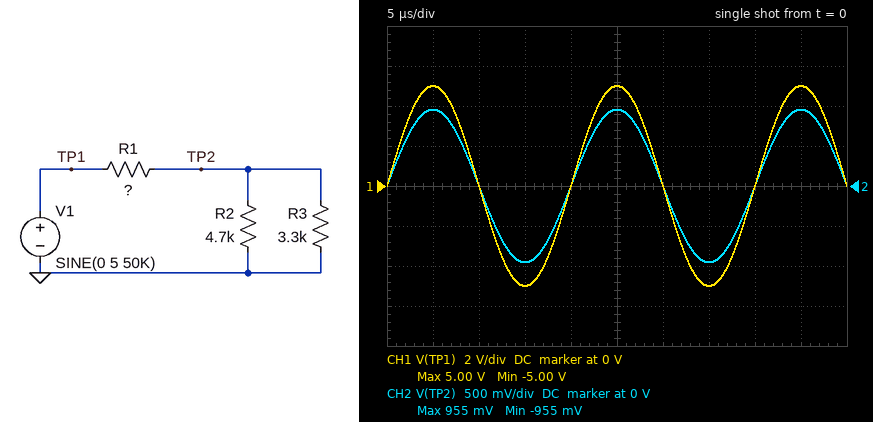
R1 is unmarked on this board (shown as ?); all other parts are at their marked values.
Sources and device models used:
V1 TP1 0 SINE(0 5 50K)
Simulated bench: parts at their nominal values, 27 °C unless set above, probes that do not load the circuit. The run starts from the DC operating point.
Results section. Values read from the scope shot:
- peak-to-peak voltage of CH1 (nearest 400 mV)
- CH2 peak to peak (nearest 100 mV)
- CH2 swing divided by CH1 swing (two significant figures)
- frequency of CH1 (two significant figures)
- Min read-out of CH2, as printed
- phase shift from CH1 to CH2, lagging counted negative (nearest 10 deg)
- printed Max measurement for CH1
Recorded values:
10.0 V
1.9 V
0.19
50 kHz
-955 mV
0 deg
5.00 V
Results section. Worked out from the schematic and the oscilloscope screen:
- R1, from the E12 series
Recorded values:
8.2 kΩ
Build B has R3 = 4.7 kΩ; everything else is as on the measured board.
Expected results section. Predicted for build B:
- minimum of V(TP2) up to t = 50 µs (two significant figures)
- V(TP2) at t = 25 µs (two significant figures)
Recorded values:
-1.1 V
1.1 V
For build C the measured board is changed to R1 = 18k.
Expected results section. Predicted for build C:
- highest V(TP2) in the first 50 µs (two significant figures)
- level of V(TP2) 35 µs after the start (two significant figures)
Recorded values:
490 mV
-490 mV
